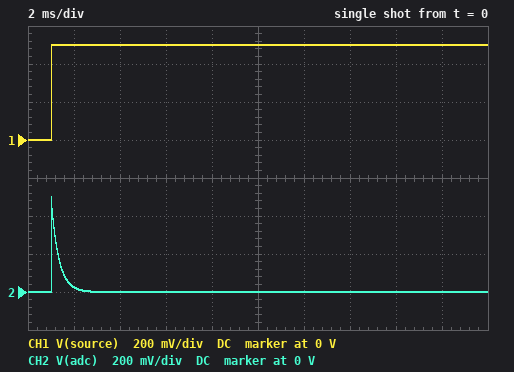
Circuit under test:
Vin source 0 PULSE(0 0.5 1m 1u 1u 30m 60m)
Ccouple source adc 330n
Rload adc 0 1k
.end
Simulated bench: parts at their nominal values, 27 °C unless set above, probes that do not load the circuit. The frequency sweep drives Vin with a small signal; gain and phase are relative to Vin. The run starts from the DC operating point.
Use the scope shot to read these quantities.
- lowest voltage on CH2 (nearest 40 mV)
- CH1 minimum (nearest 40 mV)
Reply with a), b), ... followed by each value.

a) 0 V
b) 0 V
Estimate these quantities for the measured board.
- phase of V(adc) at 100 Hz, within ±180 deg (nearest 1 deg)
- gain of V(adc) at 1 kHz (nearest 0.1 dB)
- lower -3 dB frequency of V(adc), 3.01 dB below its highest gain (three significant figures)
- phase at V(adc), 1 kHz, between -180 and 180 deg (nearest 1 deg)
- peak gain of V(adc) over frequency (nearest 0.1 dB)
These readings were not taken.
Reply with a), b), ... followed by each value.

a) 78 deg
b) -0.9 dB
c) 482 Hz
d) 26 deg
e) 0 dB
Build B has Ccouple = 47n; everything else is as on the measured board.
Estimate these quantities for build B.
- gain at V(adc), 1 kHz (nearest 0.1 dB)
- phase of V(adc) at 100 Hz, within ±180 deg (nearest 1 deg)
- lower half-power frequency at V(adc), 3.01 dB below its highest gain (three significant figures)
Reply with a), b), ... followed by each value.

a) -11.0 dB
b) 88 deg
c) 3.39 kHz
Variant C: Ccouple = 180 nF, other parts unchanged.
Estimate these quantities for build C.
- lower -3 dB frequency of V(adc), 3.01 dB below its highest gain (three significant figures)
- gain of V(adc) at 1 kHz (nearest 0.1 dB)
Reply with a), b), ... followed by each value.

a) 884 Hz
b) -2.5 dB
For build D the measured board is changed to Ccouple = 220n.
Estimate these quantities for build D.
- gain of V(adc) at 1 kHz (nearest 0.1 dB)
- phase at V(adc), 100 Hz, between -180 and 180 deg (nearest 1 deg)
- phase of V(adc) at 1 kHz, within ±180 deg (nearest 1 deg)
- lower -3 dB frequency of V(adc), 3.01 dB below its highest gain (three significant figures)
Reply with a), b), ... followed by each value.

a) -1.8 dB
b) 82 deg
c) 36 deg
d) 723 Hz
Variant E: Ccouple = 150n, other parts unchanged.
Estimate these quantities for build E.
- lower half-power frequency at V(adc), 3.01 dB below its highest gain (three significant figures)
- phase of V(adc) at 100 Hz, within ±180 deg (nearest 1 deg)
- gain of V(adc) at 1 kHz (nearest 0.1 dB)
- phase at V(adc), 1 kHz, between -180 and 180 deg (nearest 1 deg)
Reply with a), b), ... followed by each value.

a) 1.06 kHz
b) 85 deg
c) -3.3 dB
d) 47 deg
